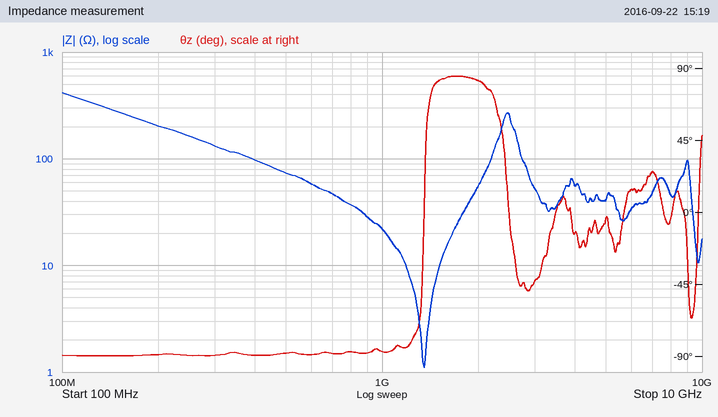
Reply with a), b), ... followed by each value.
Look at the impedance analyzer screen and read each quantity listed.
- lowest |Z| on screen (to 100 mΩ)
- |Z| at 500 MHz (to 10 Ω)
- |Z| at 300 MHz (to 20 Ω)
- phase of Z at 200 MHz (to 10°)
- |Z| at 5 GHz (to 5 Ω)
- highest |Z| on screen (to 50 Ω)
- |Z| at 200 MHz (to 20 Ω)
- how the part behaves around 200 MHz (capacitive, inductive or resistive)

a) 1.1 Ω
b) 70 Ω
c) 140 Ω
d) -90°
e) 40 Ω
f) 400 Ω
g) 200 Ω
h) capacitive
